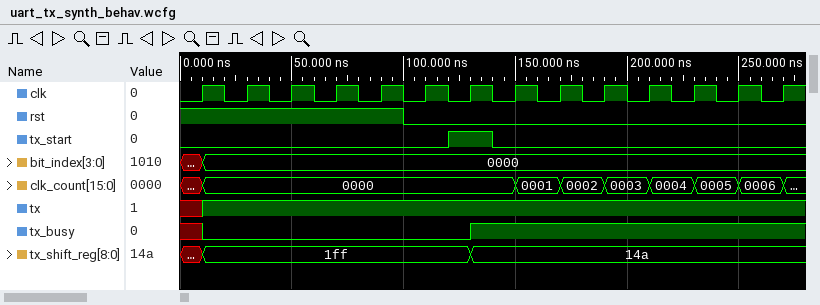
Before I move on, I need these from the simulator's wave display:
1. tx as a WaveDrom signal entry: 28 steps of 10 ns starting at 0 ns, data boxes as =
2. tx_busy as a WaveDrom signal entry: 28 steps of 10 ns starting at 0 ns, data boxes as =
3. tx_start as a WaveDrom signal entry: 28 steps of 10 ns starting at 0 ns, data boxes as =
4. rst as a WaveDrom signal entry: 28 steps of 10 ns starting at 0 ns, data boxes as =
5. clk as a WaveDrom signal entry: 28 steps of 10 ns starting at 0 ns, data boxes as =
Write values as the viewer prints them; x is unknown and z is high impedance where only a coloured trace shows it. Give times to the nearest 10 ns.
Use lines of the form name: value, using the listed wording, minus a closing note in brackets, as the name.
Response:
tx as a WaveDrom signal entry: 28 steps of 10 ns starting at 0 ns, data boxes as =: {name: 'tx', wave: 'x1..........................'}
tx_busy as a WaveDrom signal entry: 28 steps of 10 ns starting at 0 ns, data boxes as =: {name: 'tx_busy', wave: 'x0...........1..............'}
tx_start as a WaveDrom signal entry: 28 steps of 10 ns starting at 0 ns, data boxes as =: {name: 'tx_start', wave: '0...........1.0.............'}
rst as a WaveDrom signal entry: 28 steps of 10 ns starting at 0 ns, data boxes as =: {name: 'rst', wave: '1.........0.................'}
clk as a WaveDrom signal entry: 28 steps of 10 ns starting at 0 ns, data boxes as =: {name: 'clk', wave: '0101010101010101010101010101'}
